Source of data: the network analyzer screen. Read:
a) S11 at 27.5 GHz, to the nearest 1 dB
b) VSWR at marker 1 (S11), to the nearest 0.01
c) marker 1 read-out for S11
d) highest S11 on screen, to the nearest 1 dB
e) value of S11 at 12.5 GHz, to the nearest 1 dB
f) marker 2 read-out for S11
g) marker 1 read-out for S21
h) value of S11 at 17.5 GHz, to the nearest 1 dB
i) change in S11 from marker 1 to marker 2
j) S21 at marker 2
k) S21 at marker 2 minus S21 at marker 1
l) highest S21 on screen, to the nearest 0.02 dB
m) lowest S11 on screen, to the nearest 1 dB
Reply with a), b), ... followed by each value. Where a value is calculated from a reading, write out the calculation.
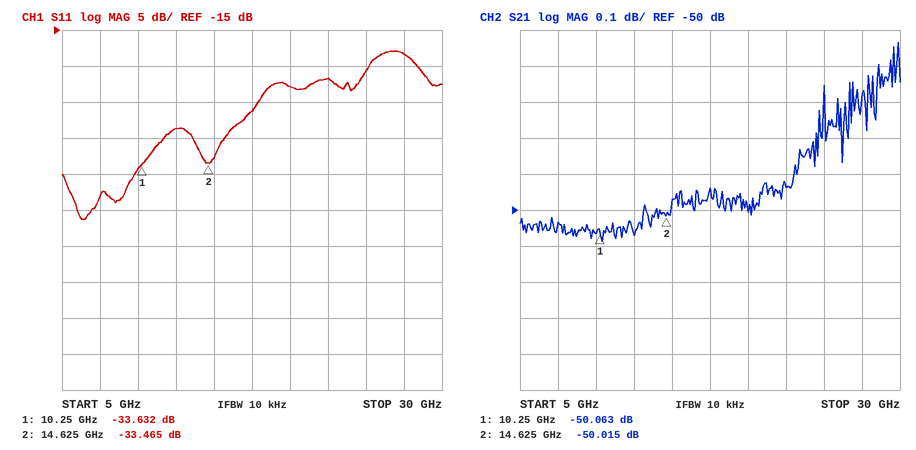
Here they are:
a) -18 dB
b) (1 + 0.0208)/(1 − 0.0208) ≈ 1.04
c) -33.632 dB
d) -18 dB
e) -29 dB
f) -33.465 dB
g) -50.063 dB
h) -26 dB
i) -33.465 − (-33.632) = 0.167 dB
j) -50.015 dB
k) -50.015 − (-50.063) = 0.048 dB
l) -49.54 dB
m) -41 dB
